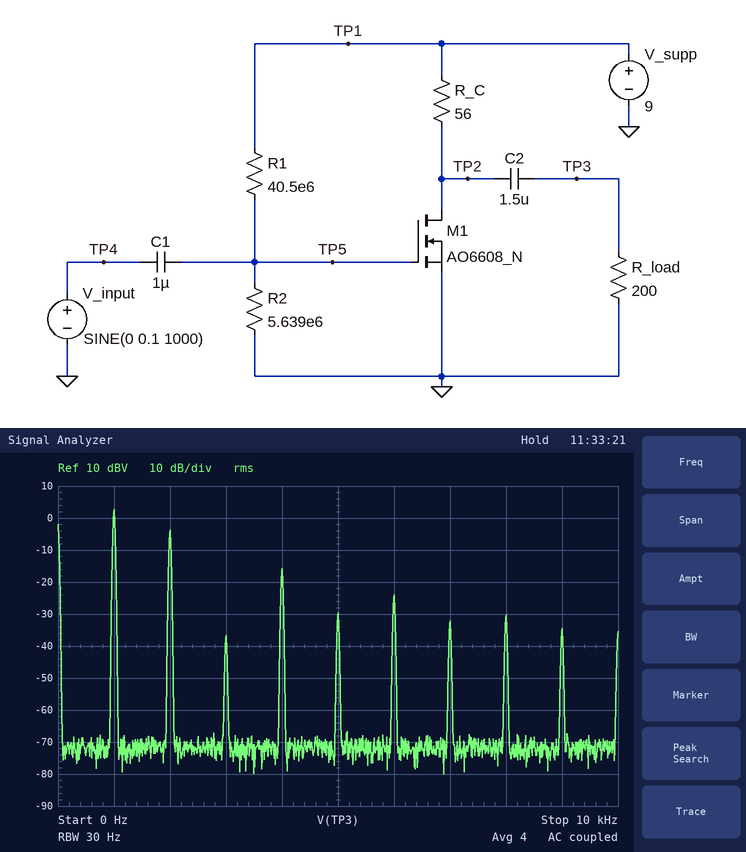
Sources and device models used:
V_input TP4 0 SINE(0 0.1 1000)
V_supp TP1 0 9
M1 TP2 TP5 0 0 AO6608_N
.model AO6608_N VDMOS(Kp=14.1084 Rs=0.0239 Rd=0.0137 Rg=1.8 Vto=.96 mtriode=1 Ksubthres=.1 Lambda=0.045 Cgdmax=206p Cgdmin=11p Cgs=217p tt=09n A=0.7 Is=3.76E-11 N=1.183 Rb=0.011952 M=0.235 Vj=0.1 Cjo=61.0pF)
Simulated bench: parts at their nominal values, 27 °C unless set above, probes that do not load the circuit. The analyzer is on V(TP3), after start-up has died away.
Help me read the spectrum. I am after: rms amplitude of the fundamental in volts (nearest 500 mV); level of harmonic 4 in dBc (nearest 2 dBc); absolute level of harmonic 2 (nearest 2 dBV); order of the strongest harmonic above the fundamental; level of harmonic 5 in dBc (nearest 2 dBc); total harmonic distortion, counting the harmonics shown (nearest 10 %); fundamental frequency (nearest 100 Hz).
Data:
1.5 V
-18 dBc
-4 dBV
2
-32 dBc
50 %
1.0 kHz
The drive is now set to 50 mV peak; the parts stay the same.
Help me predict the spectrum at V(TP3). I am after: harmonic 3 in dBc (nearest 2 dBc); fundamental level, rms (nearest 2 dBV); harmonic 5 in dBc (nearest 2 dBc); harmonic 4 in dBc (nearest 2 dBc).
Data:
-20 dBc
-4 dBV
-24 dBc
-20 dBc
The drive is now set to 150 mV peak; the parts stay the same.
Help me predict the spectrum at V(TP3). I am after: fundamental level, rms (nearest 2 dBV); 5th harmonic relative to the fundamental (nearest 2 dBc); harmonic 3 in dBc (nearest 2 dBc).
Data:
6 dBV
-42 dBc
-26 dBc
